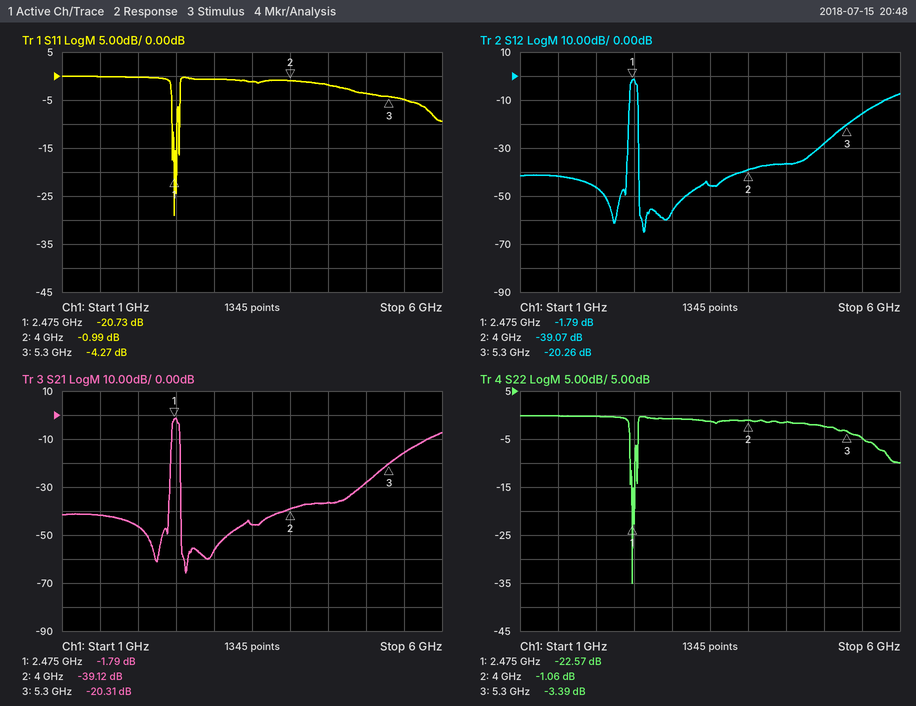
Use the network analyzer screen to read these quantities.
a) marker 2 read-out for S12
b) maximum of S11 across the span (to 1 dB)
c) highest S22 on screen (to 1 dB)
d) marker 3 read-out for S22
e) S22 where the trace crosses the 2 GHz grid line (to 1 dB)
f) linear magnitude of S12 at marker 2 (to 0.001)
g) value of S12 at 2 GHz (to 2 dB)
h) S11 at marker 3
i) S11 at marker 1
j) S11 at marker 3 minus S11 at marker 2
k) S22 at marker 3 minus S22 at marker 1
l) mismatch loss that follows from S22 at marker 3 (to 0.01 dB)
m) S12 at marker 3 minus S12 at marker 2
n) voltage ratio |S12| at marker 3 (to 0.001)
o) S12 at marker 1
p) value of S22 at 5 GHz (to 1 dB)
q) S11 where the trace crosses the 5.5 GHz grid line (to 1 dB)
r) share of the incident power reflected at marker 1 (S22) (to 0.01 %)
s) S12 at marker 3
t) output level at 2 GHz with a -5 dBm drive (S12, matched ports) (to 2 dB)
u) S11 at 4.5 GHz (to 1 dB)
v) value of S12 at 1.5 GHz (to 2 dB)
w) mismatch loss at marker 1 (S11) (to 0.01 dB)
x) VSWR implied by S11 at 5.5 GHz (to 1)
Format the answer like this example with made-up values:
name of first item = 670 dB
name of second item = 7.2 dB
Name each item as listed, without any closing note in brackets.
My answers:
marker 2 read-out for S12 = -39.07 dB
maximum of S11 across the span = 0 dB
highest S22 on screen = 0 dB
marker 3 read-out for S22 = -3.39 dB
S22 where the trace crosses the 2 GHz grid line = 0 dB
linear magnitude of S12 at marker 2 = 0.011
value of S12 at 2 GHz = -46 dB
S11 at marker 3 = -4.27 dB
S11 at marker 1 = -20.73 dB
S11 at marker 3 minus S11 at marker 2 = -3.28 dB
S22 at marker 3 minus S22 at marker 1 = 19.18 dB
mismatch loss that follows from S22 at marker 3 = 2.66 dB
S12 at marker 3 minus S12 at marker 2 = 18.81 dB
voltage ratio |S12| at marker 3 = 0.097
S12 at marker 1 = -1.79 dB
value of S22 at 5 GHz = -2 dB
S11 where the trace crosses the 5.5 GHz grid line = -5 dB
share of the incident power reflected at marker 1 (S22) = 0.55 %
S12 at marker 3 = -20.26 dB
output level at 2 GHz with a -5 dBm drive (S12, matched ports) = -52 dBm
S11 at 4.5 GHz = -2 dB
value of S12 at 1.5 GHz = -42 dB
mismatch loss at marker 1 (S11) = 0.04 dB
VSWR implied by S11 at 5.5 GHz = 4
